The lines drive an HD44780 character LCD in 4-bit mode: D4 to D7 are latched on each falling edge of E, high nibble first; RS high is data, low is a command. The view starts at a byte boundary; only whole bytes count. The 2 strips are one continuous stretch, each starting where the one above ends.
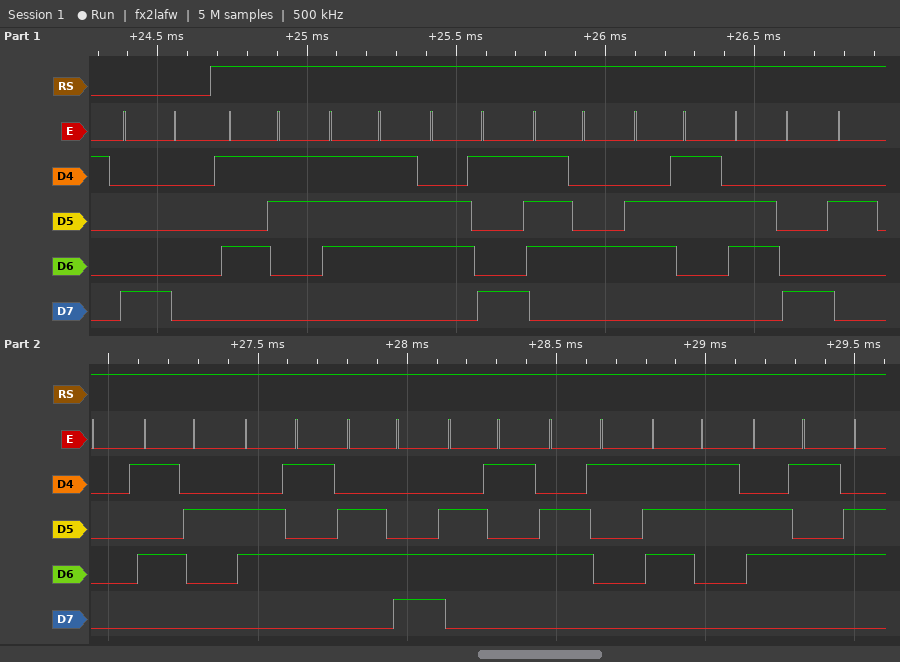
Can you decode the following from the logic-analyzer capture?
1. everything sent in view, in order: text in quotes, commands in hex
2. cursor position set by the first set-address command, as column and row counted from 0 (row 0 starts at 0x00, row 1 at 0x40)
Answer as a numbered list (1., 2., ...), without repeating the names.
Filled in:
1. 0x80 "Switch Release"
2. column 0, row 0
